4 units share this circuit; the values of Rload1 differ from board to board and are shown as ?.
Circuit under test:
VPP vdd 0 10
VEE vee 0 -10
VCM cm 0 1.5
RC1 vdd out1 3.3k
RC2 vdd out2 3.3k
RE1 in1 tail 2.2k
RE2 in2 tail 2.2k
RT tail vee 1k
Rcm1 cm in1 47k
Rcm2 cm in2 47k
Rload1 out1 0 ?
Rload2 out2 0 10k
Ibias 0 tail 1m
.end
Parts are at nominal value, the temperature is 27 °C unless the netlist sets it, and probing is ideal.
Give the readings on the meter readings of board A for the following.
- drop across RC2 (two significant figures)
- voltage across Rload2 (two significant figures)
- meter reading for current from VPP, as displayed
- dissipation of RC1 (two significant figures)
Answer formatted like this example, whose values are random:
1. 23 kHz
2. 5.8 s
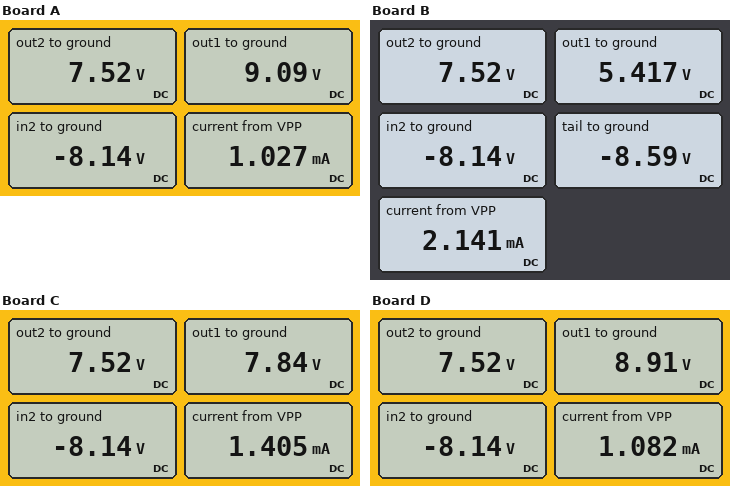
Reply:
1. 2.5 V
2. 7.5 V
3. 1.027 mA
4. 250 µW
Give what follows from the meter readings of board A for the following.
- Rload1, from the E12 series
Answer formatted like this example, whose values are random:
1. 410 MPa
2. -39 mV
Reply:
1. 33 kΩ
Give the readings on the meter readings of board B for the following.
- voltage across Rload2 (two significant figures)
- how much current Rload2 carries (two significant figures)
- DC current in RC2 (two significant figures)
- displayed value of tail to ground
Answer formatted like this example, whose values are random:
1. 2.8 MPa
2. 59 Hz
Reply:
1. 7.5 V
2. 750 µA
3. 750 µA
4. -8.59 V
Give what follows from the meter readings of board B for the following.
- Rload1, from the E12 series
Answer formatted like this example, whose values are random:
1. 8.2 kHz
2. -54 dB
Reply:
1. 3.9 kΩ
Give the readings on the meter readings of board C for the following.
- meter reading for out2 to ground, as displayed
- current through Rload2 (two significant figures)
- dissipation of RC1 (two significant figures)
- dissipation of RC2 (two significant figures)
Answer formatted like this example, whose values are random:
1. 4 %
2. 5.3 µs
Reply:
1. 7.52 V
2. 750 µA
3. 1.4 mW
4. 1.9 mW
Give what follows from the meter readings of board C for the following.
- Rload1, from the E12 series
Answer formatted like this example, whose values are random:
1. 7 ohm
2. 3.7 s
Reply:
1. 12 kΩ
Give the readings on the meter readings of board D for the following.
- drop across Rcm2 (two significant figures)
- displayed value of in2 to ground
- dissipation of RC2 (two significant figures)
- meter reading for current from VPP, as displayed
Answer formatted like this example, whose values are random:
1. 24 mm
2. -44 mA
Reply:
1. 9.6 V
2. -8.14 V
3. 1.9 mW
4. 1.082 mA
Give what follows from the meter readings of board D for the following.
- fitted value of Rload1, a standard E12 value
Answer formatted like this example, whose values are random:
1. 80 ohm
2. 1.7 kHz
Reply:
1. 27 kΩ
